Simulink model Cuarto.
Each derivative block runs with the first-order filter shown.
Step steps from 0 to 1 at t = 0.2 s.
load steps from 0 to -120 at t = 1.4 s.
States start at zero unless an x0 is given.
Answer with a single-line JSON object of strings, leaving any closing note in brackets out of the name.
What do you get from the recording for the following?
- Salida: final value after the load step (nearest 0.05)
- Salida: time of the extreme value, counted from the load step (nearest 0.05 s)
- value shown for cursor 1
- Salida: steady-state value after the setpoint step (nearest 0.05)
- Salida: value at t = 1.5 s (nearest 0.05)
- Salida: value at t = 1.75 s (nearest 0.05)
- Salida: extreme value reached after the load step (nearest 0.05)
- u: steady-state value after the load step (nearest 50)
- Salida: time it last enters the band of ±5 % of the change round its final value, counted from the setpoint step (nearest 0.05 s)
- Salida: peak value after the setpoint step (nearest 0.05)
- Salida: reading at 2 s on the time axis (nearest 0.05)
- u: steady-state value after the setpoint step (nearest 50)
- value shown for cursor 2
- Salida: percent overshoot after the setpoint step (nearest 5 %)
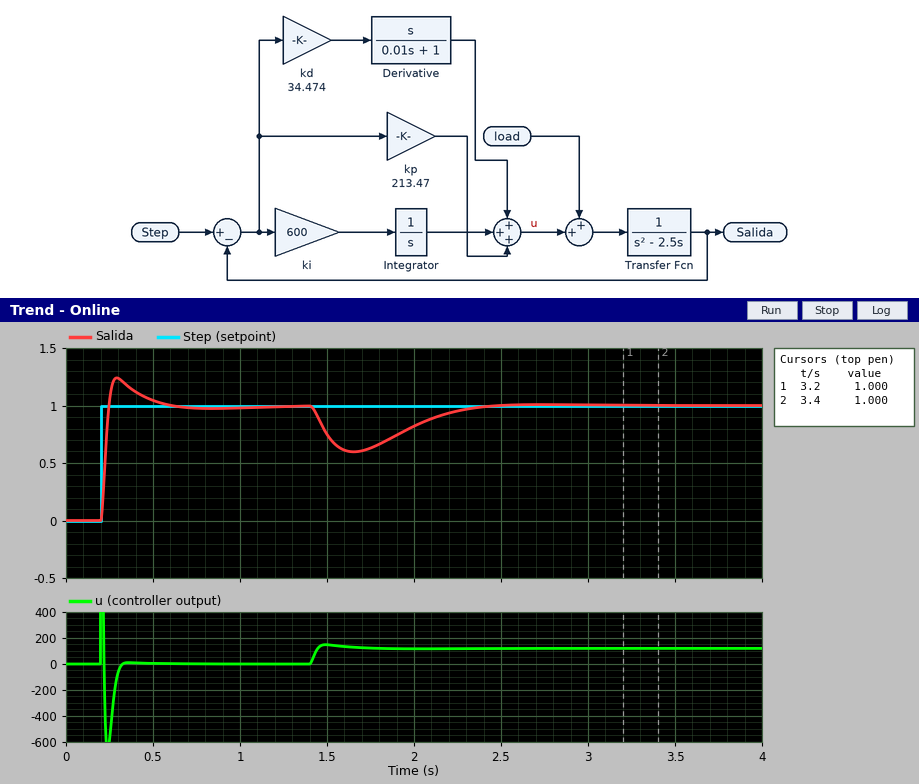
{"Salida: final value after the load step": "1.00", "Salida: time of the extreme value, counted from the load step": "0.25 s", "value shown for cursor 1": "1.000", "Salida: steady-state value after the setpoint step": "1.00", "Salida: value at t = 1.5 s": "0.75", "Salida: value at t = 1.75 s": "0.65", "Salida: extreme value reached after the load step": "0.60", "u: steady-state value after the load step": "100", "Salida: time it last enters the band of ±5 % of the change round its final value, counted from the setpoint step": "0.30 s", "Salida: peak value after the setpoint step": "1.25", "Salida: reading at 2 s on the time axis": "0.80", "u: steady-state value after the setpoint step": "0", "value shown for cursor 2": "1.000", "Salida: percent overshoot after the setpoint step": "25 %"}
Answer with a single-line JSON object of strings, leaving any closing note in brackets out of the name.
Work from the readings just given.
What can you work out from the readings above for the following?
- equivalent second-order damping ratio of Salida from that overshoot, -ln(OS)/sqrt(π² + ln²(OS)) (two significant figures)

{"equivalent second-order damping ratio of Salida from that overshoot, -ln(OS)/sqrt(π² + ln²(OS))": "0.40"}
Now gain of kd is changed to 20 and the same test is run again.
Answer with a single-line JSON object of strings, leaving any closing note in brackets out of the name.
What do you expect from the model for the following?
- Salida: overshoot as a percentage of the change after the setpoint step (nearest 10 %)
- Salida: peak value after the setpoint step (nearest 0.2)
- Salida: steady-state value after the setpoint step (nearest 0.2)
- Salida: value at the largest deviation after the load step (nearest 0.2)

{"Salida: overshoot as a percentage of the change after the setpoint step": "40 %", "Salida: peak value after the setpoint step": "1.4", "Salida: steady-state value after the setpoint step": "1.0", "Salida: value at the largest deviation after the load step": "0.4"}
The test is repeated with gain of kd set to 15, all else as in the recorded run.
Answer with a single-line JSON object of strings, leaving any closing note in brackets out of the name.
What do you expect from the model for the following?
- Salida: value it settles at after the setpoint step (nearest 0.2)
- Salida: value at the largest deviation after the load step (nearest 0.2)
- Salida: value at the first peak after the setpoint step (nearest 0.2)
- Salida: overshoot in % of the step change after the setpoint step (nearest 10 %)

{"Salida: value it settles at after the setpoint step": "1.0", "Salida: value at the largest deviation after the load step": "0.4", "Salida: value at the first peak after the setpoint step": "1.6", "Salida: overshoot in % of the step change after the setpoint step": "50 %"}
